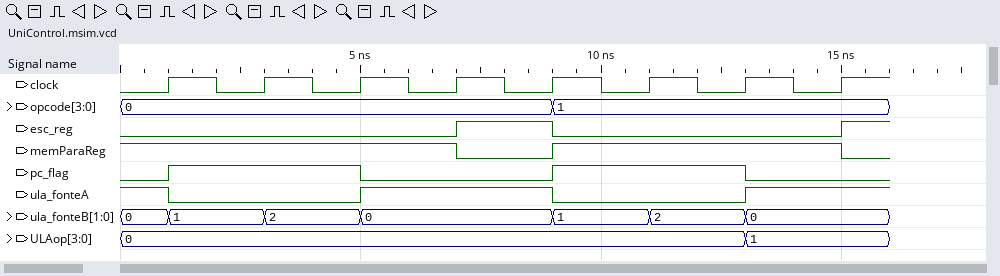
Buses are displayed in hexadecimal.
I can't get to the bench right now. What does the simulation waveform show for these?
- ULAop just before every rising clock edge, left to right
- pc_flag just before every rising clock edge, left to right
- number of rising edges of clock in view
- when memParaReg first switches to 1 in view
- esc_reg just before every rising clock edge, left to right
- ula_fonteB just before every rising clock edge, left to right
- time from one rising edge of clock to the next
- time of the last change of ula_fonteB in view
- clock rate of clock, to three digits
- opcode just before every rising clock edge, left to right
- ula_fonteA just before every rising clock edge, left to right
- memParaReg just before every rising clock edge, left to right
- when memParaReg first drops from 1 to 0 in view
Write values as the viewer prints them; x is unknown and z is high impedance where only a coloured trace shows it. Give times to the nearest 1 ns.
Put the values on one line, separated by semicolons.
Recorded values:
0, 0, 0, 0, 0, 0, 0, 1; 0 1 1 0 0 1 1 0; 8; 9 ns; 0 0 0 0 1 0 0 0; 0, 1, 2, 0, 0, 1, 2, 0; 2 ns; 13 ns; 500 MHz; 0, 0, 0, 0, 0, 1, 1, 1; 1 0 0 1 1 0 0 1; 1 1 1 1 0 1 1 1; 7 ns
